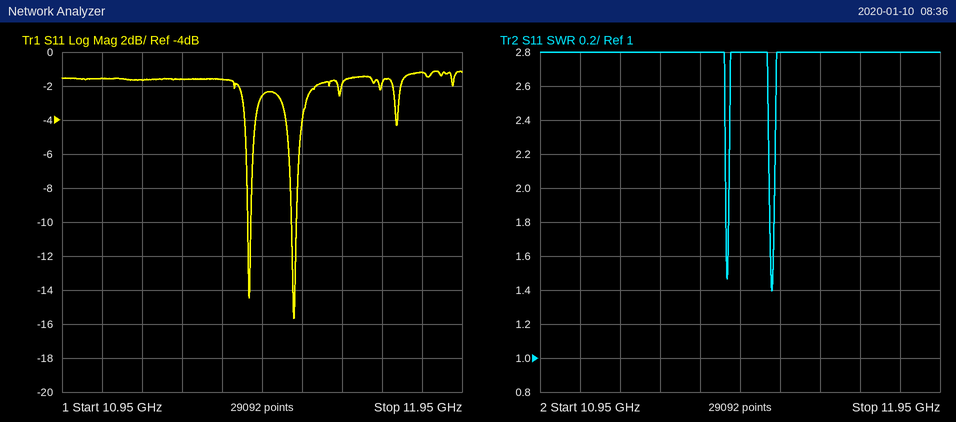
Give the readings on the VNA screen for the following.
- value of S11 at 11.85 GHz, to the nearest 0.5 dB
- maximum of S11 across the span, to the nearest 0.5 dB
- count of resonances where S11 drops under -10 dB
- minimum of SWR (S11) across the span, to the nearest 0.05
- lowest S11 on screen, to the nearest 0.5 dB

-1.0 dB
-1.0 dB
2
1.40
-15.5 dB
